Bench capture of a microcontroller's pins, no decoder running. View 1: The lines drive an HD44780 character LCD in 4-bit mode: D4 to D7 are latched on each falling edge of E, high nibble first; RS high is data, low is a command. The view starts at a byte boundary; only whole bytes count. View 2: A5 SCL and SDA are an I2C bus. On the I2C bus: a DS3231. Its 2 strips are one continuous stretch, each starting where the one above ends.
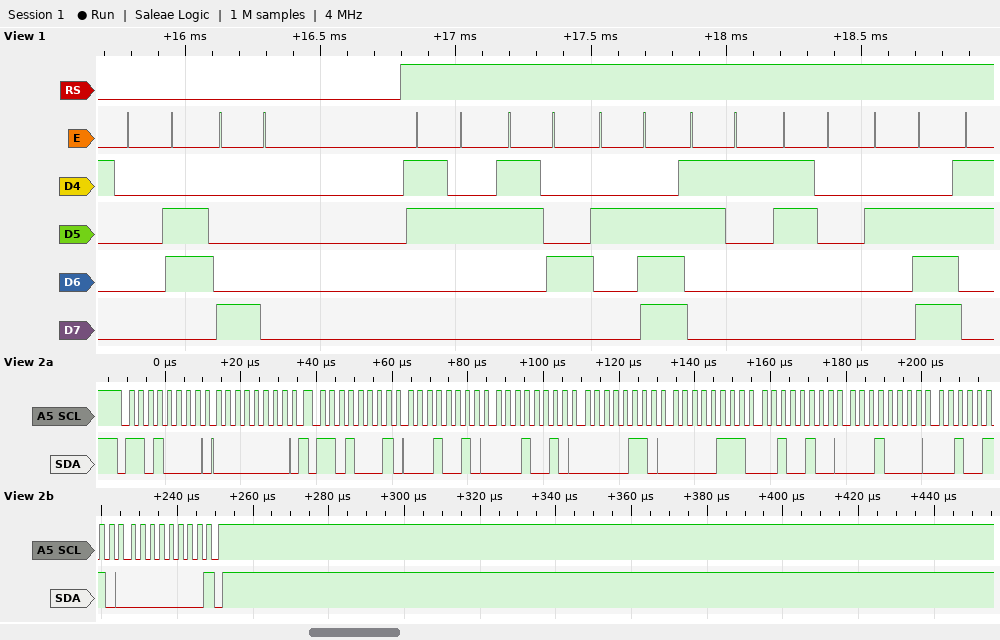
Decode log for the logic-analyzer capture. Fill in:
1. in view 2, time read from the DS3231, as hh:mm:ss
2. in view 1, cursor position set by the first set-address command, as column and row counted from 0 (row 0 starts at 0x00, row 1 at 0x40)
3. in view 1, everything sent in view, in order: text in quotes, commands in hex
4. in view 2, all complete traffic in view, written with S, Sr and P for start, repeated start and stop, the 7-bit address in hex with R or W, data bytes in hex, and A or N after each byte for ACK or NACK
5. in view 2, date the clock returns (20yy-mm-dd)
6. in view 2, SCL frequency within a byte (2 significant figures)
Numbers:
06:12:12
column 0, row 0
0x06 0x80 "24.10."
S 68W A 00 A Sr 68R A 12 A 12 A 06 A 07 A 24 A 10 A 26 A 00 N P
2026-10-24
400 kHz
